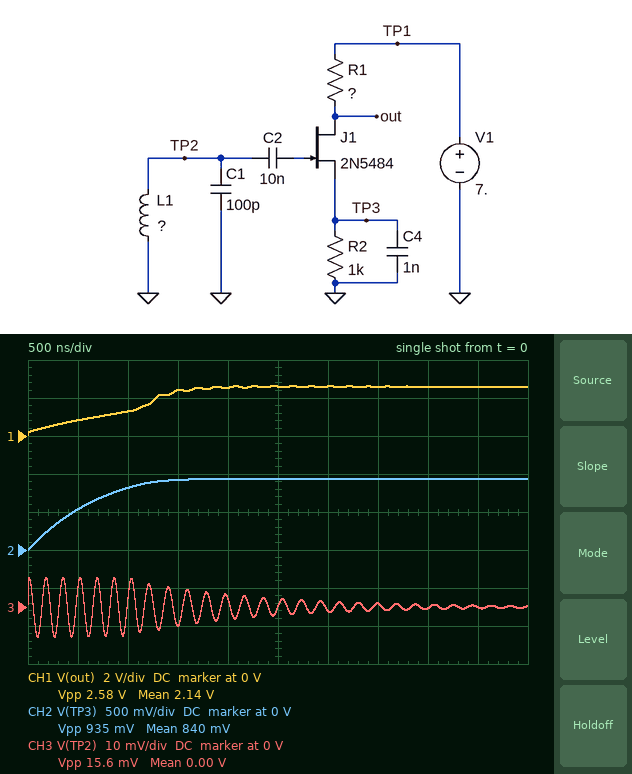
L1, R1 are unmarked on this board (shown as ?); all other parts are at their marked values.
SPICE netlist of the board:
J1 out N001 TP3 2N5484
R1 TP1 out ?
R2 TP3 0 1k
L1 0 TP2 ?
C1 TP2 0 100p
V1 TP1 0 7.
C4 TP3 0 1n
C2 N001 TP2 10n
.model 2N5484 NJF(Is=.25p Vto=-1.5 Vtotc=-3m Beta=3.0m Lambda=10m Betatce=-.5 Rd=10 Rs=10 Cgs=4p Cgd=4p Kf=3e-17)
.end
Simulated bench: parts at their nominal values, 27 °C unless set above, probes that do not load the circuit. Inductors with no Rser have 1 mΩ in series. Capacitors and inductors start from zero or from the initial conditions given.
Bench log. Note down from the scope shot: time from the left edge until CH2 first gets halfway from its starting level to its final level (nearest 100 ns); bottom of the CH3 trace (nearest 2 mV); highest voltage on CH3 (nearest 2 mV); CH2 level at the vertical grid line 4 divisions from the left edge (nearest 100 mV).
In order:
400 ns
-8 mV
8 mV
900 mV
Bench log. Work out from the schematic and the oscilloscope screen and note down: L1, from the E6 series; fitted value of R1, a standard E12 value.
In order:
6.8 µH
4.7 kΩ
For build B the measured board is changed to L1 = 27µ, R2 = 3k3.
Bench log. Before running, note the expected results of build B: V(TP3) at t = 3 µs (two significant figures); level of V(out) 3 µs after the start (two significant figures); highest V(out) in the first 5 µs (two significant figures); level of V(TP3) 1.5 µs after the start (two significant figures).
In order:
1.2 V
5.3 V
5.5 V
1.1 V
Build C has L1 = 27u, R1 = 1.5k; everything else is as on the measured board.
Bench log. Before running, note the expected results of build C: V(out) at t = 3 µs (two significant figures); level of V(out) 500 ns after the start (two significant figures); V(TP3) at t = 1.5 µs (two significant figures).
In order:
5.8 V
5.1 V
950 mV
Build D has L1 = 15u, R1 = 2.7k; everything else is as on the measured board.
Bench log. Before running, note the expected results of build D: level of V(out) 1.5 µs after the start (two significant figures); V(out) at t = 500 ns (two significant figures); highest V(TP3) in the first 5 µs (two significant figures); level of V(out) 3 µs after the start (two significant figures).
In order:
4.5 V
3.1 V
940 mV
4.4 V
